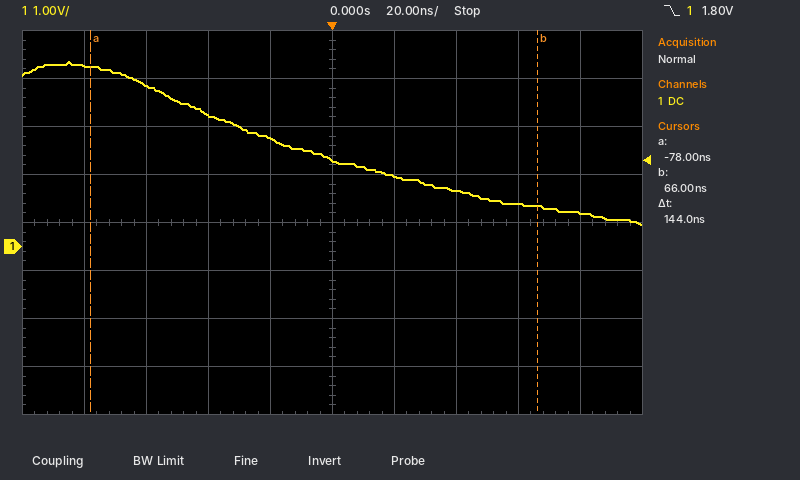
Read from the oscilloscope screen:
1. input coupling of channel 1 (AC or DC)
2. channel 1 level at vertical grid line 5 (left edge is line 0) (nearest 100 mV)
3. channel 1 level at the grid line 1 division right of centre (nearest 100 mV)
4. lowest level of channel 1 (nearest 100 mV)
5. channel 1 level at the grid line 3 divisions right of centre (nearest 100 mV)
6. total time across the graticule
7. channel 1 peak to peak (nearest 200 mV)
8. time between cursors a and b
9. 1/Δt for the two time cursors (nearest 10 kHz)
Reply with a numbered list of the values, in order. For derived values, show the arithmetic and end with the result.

1. DC
2. 1.8 V
3. 1.5 V
4. 500 mV
5. 900 mV
6. 200 ns
7. 3.4 V
8. 144 ns
9. 1 / 144 ns ≈ 6.94 MHz
